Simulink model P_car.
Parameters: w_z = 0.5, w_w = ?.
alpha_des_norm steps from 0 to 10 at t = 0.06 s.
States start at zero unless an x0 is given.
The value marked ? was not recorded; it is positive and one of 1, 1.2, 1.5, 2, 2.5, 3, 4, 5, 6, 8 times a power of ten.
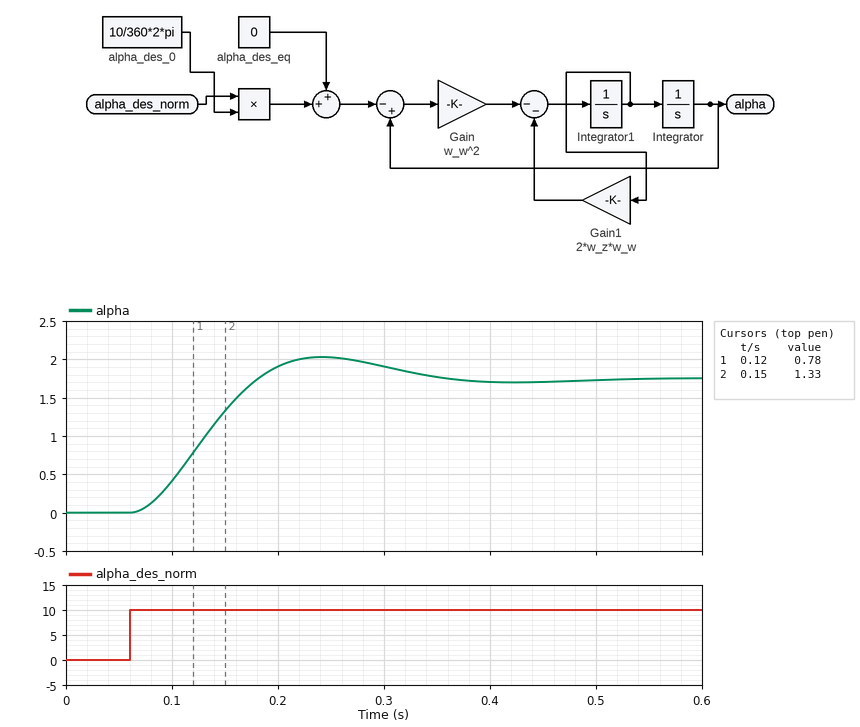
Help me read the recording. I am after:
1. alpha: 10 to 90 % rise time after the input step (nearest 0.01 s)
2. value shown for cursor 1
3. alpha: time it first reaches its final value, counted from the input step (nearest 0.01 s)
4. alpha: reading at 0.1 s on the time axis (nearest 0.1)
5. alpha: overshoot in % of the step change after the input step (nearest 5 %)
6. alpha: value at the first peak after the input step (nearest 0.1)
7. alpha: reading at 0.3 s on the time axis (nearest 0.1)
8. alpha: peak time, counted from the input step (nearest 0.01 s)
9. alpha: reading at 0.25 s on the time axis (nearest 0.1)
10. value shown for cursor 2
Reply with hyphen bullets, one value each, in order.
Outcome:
- 0.08 s
- 0.78
- 0.12 s
- 0.4
- 15 %
- 2.0
- 1.9
- 0.18 s
- 2.0
- 1.33
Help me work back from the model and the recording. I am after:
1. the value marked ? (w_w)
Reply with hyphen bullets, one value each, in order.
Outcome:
- 20
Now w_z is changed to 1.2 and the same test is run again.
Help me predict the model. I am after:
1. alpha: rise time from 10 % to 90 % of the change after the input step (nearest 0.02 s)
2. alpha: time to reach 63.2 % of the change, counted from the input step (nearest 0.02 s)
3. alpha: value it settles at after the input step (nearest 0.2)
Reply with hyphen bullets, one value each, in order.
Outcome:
- 0.22 s
- 0.12 s
- 1.8
